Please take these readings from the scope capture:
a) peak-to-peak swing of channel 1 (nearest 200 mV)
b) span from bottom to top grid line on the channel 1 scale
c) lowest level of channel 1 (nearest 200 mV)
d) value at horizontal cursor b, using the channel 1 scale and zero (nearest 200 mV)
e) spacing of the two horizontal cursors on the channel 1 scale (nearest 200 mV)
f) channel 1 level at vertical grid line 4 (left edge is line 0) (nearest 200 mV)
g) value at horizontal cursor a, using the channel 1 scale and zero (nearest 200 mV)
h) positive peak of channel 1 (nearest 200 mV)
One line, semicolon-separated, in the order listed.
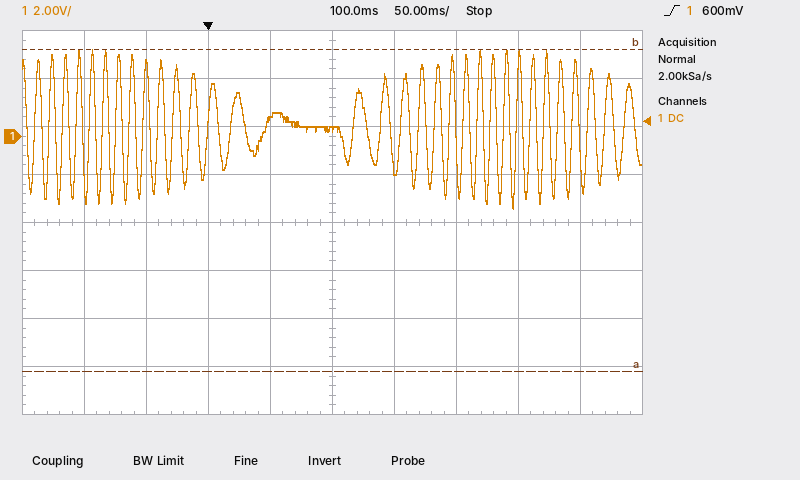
6.6 V; 16 V; -3.0 V; 3.6 V; 13.4 V; 800 mV; -9.8 V; 3.6 V
